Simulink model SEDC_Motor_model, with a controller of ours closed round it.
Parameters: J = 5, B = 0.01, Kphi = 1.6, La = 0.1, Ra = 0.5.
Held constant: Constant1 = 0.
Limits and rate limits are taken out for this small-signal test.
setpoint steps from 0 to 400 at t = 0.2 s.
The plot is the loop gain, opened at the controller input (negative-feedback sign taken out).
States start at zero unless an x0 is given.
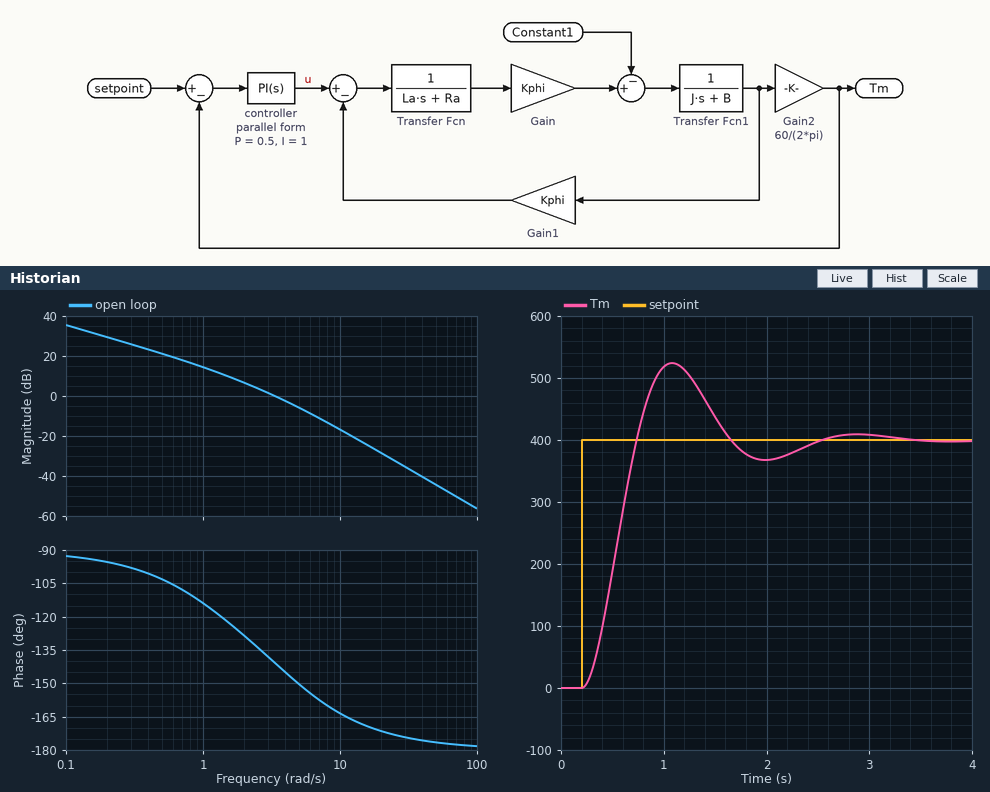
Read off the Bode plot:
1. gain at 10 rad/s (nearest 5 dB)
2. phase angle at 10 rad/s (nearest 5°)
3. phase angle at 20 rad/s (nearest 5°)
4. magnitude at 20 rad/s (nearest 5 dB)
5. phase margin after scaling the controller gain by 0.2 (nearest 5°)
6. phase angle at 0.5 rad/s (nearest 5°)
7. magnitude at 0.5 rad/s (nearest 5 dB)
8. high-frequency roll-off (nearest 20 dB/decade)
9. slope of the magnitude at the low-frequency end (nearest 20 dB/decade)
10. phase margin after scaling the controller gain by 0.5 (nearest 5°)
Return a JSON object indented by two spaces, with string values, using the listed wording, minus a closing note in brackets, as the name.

{
  "gain at 10 rad/s": "-15 dB",
  "phase angle at 10 rad/s": "-165°",
  "phase angle at 20 rad/s": "-170°",
  "magnitude at 20 rad/s": "-30 dB",
  "phase margin after scaling the controller gain by 0.2": "65°",
  "phase angle at 0.5 rad/s": "-105°",
  "magnitude at 0.5 rad/s": "20 dB",
  "high-frequency roll-off": "-40 dB/decade",
  "slope of the magnitude at the low-frequency end": "-20 dB/decade",
  "phase margin after scaling the controller gain by 0.5": "50°"
}
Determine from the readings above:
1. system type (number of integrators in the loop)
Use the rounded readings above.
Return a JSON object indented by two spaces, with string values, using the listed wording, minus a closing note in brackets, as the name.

{
  "system type": "1"
}
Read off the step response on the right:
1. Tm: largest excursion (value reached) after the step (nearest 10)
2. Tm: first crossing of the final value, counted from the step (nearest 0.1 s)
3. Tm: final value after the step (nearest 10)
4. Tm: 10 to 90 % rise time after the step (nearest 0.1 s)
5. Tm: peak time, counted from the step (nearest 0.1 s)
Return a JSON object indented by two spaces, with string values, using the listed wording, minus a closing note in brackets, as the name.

{
  "Tm: largest excursion (value reached) after the step": "520",
  "Tm: first crossing of the final value, counted from the step": "0.5 s",
  "Tm: final value after the step": "400",
  "Tm: 10 to 90 % rise time after the step": "0.4 s",
  "Tm: peak time, counted from the step": "0.9 s"
}
